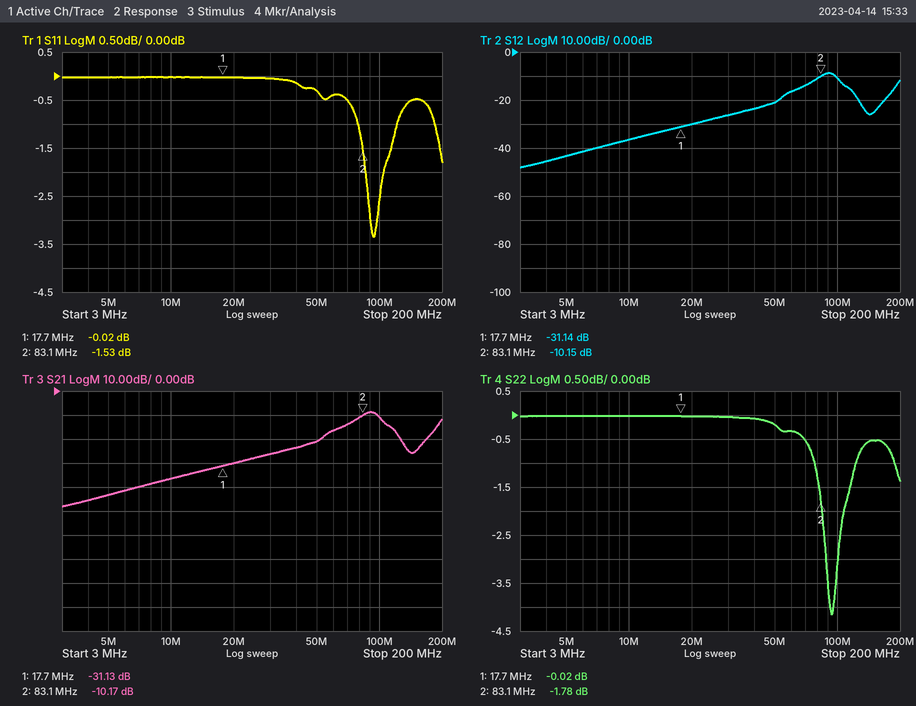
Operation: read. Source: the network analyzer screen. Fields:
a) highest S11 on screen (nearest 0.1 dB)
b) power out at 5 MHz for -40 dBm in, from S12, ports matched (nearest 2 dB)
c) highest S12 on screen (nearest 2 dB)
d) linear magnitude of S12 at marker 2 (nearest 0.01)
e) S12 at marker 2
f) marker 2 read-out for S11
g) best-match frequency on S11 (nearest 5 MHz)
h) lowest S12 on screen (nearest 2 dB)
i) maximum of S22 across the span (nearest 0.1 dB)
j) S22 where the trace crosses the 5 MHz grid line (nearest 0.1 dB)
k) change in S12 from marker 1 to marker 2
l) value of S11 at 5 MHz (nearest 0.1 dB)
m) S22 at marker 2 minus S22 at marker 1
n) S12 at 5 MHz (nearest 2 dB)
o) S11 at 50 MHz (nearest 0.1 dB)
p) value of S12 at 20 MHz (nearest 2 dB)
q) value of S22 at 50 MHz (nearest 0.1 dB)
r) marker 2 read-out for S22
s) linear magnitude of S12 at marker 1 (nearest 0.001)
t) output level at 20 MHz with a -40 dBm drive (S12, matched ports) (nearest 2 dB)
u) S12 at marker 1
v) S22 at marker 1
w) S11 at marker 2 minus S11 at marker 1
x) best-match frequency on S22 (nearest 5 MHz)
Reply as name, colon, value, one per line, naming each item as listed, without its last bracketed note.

highest S11 on screen: 0.0 dB
power out at 5 MHz for -40 dBm in, from S12, ports matched: -84 dBm
highest S12 on screen: -8 dB
linear magnitude of S12 at marker 2: 0.31
S12 at marker 2: -10.15 dB
marker 2 read-out for S11: -1.53 dB
best-match frequency on S11: 95 MHz
lowest S12 on screen: -48 dB
maximum of S22 across the span: 0.0 dB
S22 where the trace crosses the 5 MHz grid line: 0.0 dB
change in S12 from marker 1 to marker 2: 20.99 dB
value of S11 at 5 MHz: 0.0 dB
S22 at marker 2 minus S22 at marker 1: -1.76 dB
S12 at 5 MHz: -44 dB
S11 at 50 MHz: -0.3 dB
value of S12 at 20 MHz: -30 dB
value of S22 at 50 MHz: -0.2 dB
marker 2 read-out for S22: -1.78 dB
linear magnitude of S12 at marker 1: 0.028
output level at 20 MHz with a -40 dBm drive (S12, matched ports): -70 dBm
S12 at marker 1: -31.14 dB
S22 at marker 1: -0.02 dB
S11 at marker 2 minus S11 at marker 1: -1.51 dB
best-match frequency on S22: 95 MHz
